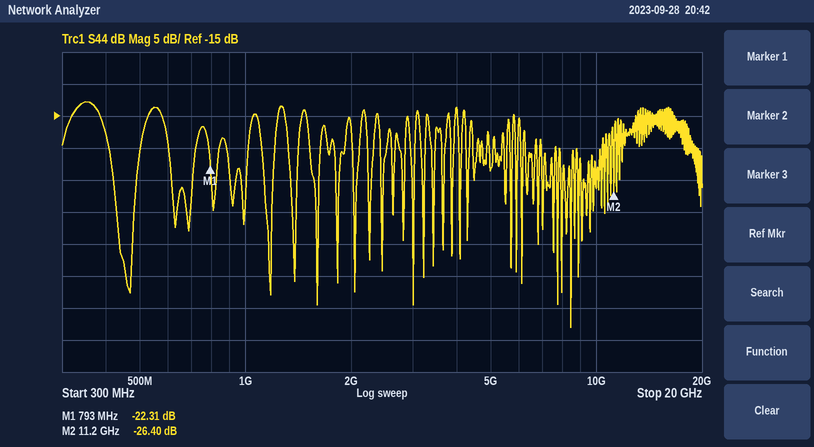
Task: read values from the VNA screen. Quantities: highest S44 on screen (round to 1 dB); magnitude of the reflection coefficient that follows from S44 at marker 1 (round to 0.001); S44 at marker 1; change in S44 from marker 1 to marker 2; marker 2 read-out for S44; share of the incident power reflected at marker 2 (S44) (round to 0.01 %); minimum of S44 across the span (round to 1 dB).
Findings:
-13 dB
0.077
-22.31 dB
-4.09 dB
-26.40 dB
0.23 %
-48 dB
